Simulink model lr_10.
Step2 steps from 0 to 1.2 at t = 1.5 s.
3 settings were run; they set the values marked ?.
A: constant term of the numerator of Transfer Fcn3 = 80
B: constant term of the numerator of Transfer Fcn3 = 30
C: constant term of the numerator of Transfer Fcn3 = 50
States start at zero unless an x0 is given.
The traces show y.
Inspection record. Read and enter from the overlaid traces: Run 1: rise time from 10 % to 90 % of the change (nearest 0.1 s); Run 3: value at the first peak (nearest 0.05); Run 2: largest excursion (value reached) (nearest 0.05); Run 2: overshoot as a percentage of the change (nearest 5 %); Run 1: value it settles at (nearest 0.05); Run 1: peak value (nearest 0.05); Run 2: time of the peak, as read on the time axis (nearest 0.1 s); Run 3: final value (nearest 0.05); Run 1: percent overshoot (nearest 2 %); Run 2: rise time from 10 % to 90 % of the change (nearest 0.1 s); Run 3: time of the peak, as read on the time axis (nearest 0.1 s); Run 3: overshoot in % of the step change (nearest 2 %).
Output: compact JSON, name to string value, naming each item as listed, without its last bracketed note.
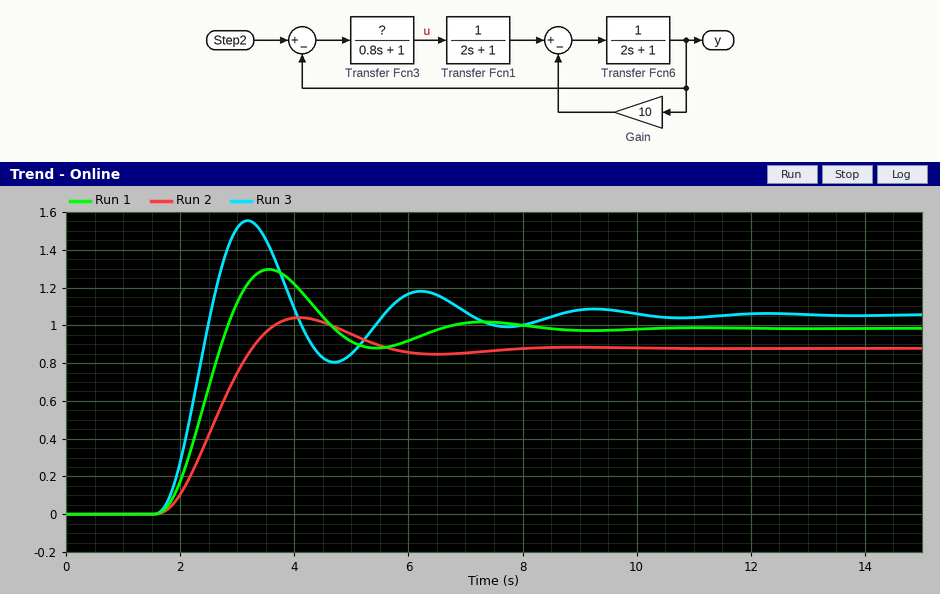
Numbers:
{"Run 1: rise time from 10 % to 90 % of the change": "0.8 s", "Run 3: value at the first peak": "1.55", "Run 2: largest excursion (value reached)": "1.05", "Run 2: overshoot as a percentage of the change": "20 %", "Run 1: value it settles at": "1.00", "Run 1: peak value": "1.30", "Run 2: time of the peak, as read on the time axis": "4.1 s", "Run 3: final value": "1.05", "Run 1: percent overshoot": "32 %", "Run 2: rise time from 10 % to 90 % of the change": "1.1 s", "Run 3: time of the peak, as read on the time axis": "3.2 s", "Run 3: overshoot in % of the step change": "48 %"}
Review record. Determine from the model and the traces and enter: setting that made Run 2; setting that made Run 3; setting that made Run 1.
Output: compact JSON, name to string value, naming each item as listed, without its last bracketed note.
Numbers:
{"setting that made Run 2": "B", "setting that made Run 3": "A", "setting that made Run 1": "C"}
